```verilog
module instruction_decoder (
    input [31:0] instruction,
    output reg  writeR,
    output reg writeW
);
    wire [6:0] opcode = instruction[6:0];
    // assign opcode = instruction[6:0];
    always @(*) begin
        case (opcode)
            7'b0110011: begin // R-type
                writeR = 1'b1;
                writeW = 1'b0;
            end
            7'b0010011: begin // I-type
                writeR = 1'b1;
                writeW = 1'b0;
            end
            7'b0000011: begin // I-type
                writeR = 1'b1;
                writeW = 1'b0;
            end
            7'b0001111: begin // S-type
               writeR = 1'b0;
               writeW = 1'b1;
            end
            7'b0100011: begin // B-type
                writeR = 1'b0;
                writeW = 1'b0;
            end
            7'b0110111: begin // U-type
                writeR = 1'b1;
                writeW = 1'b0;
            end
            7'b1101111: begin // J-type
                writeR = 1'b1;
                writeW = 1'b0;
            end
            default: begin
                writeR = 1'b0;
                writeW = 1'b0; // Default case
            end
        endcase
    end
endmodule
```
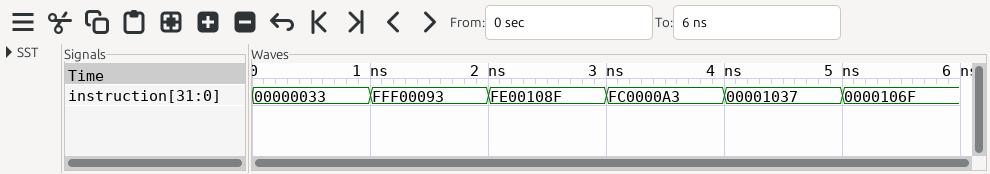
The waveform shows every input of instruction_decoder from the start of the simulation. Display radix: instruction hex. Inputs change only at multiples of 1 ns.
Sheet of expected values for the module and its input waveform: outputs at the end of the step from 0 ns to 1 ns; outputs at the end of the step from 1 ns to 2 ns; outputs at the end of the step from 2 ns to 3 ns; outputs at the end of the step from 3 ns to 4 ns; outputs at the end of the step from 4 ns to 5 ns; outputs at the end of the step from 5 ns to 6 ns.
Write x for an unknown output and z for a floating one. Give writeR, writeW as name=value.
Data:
writeR=1, writeW=0
writeR=1, writeW=0
writeR=0, writeW=1
writeR=0, writeW=0
writeR=1, writeW=0
writeR=1, writeW=0
